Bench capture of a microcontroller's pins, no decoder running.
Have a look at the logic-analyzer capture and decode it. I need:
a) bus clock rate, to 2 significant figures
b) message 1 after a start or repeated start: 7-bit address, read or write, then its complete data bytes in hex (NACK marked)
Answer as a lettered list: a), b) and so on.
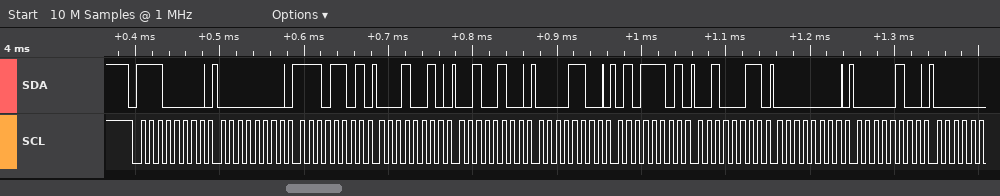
a) 100 kHz
b) 0x70 write: 00 ED 12 24 0C 5D 23 00 04
